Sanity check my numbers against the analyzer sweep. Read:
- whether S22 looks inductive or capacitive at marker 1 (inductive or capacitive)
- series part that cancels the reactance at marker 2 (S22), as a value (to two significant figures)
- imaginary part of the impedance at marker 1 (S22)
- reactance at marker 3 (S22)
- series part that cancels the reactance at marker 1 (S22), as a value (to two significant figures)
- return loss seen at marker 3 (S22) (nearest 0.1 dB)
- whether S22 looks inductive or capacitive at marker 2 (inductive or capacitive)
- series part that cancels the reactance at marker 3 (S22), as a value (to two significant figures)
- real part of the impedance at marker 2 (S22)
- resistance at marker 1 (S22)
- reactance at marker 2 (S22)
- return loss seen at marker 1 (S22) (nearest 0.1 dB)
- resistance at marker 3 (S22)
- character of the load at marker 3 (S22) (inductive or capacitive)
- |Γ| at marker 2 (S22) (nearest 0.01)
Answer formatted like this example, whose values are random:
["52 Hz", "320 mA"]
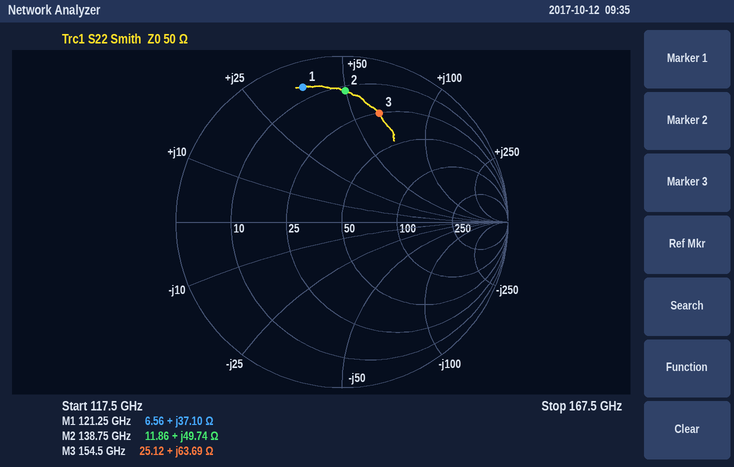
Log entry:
["inductive", "23 fF", "+37.10 Ω", "+63.69 Ω", "35 fF", "3.2 dB", "inductive", "16 fF", "11.86 Ω", "6.56 Ω", "+49.74 Ω", "1.5 dB", "25.12 Ω", "inductive", "0.79"]
